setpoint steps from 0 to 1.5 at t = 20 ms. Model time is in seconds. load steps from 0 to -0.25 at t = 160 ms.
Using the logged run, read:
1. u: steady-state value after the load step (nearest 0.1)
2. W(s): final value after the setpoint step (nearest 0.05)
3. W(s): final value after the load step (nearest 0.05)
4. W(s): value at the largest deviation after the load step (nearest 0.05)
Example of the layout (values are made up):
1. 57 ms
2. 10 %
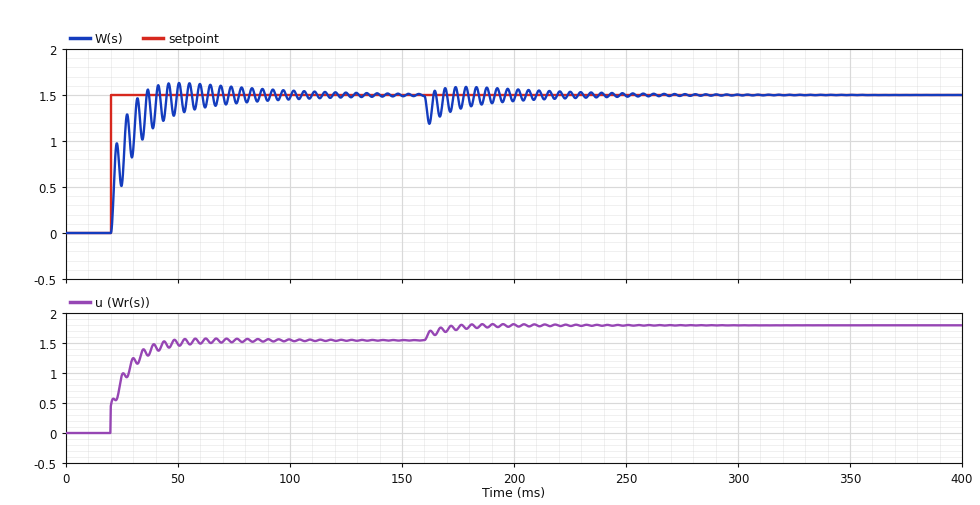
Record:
1. 1.8
2. 1.50
3. 1.50
4. 1.20
